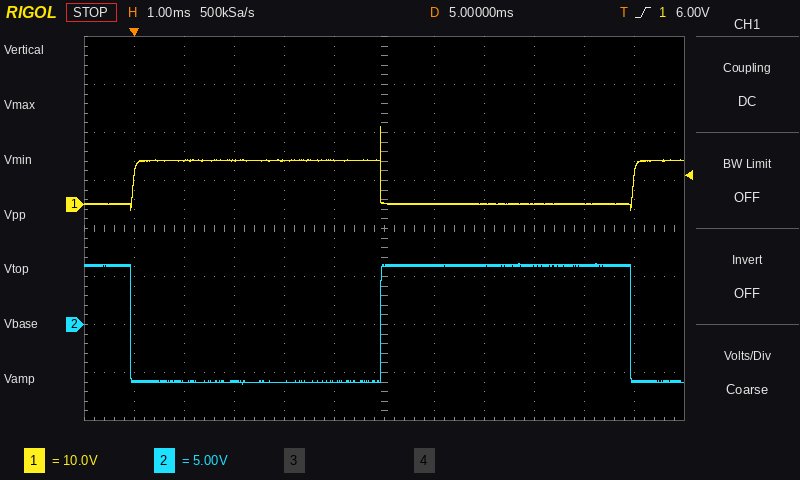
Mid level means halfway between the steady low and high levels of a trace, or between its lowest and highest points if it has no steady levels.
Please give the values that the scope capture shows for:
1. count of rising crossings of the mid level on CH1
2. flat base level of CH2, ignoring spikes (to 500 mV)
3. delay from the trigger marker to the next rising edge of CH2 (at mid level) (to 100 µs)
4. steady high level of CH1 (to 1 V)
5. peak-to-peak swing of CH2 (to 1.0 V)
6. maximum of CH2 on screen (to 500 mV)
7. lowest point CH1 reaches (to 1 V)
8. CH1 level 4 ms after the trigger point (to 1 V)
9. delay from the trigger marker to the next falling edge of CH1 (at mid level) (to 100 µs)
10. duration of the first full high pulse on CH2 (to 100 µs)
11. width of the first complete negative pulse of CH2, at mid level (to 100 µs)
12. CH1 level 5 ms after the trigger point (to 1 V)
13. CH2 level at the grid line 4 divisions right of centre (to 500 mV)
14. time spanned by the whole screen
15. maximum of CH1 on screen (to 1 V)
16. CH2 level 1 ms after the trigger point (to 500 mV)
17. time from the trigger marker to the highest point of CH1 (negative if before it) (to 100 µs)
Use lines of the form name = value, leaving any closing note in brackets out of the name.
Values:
count of rising crossings of the mid level on CH1 = 2
flat base level of CH2, ignoring spikes = -6.0 V
delay from the trigger marker to the next rising edge of CH2 (at mid level) = 4.9 ms
steady high level of CH1 = 9 V
peak-to-peak swing of CH2 = 13.0 V
maximum of CH2 on screen = 6.5 V
lowest point CH1 reaches = -1 V
CH1 level 4 ms after the trigger point = 9 V
delay from the trigger marker to the next falling edge of CH1 (at mid level) = 4.9 ms
duration of the first full high pulse on CH2 = 5.0 ms
width of the first complete negative pulse of CH2, at mid level = 5.0 ms
CH1 level 5 ms after the trigger point = 0 V
CH2 level at the grid line 4 divisions right of centre = 6.0 V
time spanned by the whole screen = 12 ms
maximum of CH1 on screen = 16 V
CH2 level 1 ms after the trigger point = -6.0 V
time from the trigger marker to the highest point of CH1 (negative if before it) = +4.9 ms
